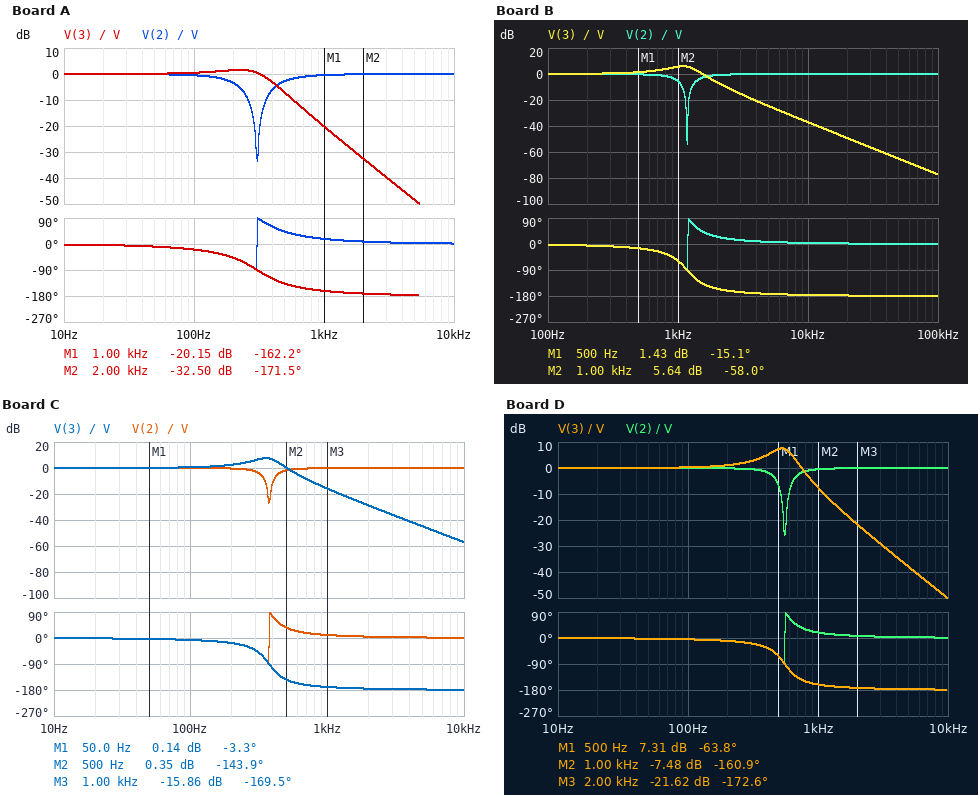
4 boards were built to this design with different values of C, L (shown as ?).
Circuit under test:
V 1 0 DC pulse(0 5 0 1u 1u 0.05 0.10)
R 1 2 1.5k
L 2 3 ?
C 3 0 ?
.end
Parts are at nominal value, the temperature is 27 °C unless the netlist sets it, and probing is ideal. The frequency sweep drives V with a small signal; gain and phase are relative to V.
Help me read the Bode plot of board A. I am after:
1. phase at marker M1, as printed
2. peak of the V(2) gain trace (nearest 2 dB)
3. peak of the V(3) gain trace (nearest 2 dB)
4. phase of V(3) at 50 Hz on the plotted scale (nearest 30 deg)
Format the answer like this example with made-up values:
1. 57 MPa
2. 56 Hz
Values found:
1. -162.2 deg
2. 0 dB
3. 2 dB
4. 0 deg
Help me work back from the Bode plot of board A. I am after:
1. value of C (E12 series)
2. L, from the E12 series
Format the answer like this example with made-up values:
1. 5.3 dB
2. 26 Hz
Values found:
1. 330 nF
2. 820 mH
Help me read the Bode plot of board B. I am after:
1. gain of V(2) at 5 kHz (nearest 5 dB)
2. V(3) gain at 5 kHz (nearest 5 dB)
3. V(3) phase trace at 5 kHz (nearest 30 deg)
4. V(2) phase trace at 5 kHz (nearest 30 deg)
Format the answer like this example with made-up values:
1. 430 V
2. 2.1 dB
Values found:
1. 0 dB
2. -25 dB
3. -180 deg
4. 0 deg
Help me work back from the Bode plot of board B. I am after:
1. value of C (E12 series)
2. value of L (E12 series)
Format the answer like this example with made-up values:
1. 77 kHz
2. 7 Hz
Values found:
1. 47 nF
2. 390 mH
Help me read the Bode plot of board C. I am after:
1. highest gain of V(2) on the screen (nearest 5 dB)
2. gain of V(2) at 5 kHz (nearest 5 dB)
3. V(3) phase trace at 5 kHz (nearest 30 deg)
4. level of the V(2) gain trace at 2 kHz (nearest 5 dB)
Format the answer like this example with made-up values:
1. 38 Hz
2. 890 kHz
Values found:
1. 0 dB
2. 0 dB
3. -180 deg
4. 0 dB
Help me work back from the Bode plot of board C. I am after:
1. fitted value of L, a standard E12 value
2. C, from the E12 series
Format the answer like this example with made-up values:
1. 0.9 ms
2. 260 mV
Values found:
1. 1.5 H
2. 120 nF
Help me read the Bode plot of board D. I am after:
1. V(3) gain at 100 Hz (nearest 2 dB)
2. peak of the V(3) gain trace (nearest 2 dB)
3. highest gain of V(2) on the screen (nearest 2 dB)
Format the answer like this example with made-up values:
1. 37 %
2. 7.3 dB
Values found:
1. 0 dB
2. 8 dB
3. 0 dB
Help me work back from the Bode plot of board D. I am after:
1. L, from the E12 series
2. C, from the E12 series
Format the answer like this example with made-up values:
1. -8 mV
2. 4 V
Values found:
1. 1 H
2. 82 nF
